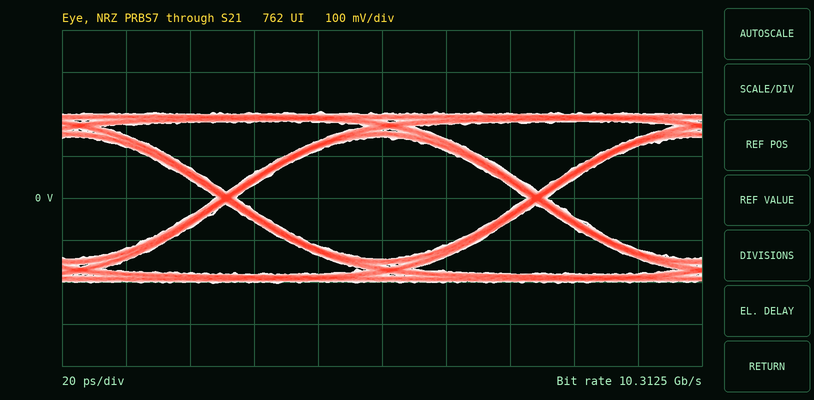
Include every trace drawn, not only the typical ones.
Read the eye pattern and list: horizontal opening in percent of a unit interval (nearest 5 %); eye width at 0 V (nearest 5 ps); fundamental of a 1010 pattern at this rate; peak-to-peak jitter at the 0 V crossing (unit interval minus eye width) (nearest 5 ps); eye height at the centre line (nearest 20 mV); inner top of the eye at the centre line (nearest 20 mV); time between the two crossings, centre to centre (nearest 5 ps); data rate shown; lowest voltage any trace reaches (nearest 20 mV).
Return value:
95 %
90 ps
5.15625 GHz
5 ps
300 mV
140 mV
95 ps
10.3125 Gb/s
-200 mV
